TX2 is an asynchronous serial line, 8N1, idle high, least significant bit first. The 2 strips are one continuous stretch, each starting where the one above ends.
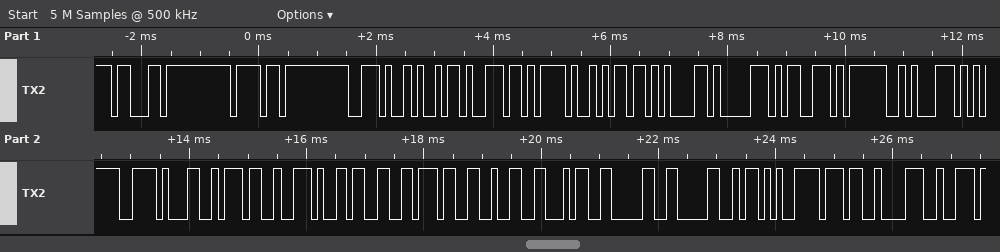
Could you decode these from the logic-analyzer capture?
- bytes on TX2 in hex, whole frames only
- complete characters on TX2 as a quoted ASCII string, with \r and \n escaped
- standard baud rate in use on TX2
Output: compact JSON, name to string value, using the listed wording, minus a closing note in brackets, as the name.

{"bytes on TX2 in hex, whole frames only": "63 6F 2E 69 6E 2F 6D 61 70 73 3F 71 3D 31 37 2E 33 37 32 34 30 30 2B 37 38", "complete characters on TX2 as a quoted ASCII string, with \\r and \\n escaped": "\"co.in/maps?q=17.372400+78\"", "standard baud rate in use on TX2": "9600 baud"}
